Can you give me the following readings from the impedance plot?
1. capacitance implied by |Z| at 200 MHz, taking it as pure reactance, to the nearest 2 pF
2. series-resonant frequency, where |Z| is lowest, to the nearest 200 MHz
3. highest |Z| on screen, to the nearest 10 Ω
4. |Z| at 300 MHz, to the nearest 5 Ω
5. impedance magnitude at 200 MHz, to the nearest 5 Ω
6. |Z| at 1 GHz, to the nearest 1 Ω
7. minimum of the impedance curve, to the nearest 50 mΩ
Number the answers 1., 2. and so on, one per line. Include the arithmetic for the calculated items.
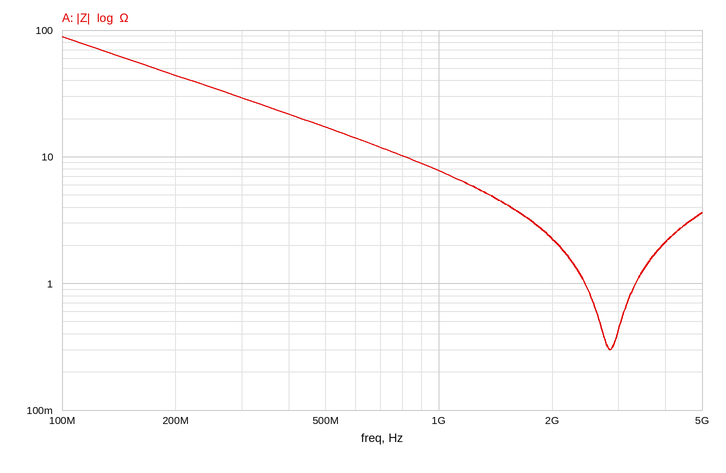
1. C = 1/(2π × 200 MHz × 45 Ω) ≈ 18 pF
2. 2.8 GHz
3. 90 Ω
4. 30 Ω
5. 45 Ω
6. 8 Ω
7. 300 mΩ
